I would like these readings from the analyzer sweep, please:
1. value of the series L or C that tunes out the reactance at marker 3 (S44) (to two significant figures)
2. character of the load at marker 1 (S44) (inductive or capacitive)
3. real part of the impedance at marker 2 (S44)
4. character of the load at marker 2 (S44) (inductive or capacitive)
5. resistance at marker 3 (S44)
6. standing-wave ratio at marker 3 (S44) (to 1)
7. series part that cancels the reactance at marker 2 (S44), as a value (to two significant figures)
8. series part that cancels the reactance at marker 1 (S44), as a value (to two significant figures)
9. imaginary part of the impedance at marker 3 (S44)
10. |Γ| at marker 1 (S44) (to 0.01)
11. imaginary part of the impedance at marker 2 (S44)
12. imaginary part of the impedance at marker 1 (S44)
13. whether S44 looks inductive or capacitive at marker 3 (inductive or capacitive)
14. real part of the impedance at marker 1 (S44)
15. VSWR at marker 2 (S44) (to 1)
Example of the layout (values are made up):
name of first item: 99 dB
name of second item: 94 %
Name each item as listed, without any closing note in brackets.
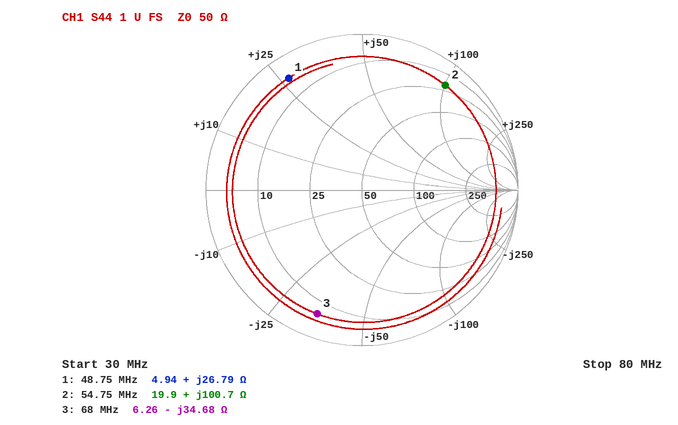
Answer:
value of the series L or C that tunes out the reactance at marker 3 (S44): 81 nH
character of the load at marker 1 (S44): inductive
real part of the impedance at marker 2: 19.9 Ω
character of the load at marker 2 (S44): inductive
resistance at marker 3: 6.26 Ω
standing-wave ratio at marker 3 (S44): 12
series part that cancels the reactance at marker 2 (S44), as a value: 29 pF
series part that cancels the reactance at marker 1 (S44), as a value: 120 pF
imaginary part of the impedance at marker 3: -34.68 Ω
|Γ| at marker 1 (S44): 0.86
imaginary part of the impedance at marker 2: +100.7 Ω
imaginary part of the impedance at marker 1: +26.79 Ω
whether S44 looks inductive or capacitive at marker 3: capacitive
real part of the impedance at marker 1: 4.94 Ω
VSWR at marker 2 (S44): 13
